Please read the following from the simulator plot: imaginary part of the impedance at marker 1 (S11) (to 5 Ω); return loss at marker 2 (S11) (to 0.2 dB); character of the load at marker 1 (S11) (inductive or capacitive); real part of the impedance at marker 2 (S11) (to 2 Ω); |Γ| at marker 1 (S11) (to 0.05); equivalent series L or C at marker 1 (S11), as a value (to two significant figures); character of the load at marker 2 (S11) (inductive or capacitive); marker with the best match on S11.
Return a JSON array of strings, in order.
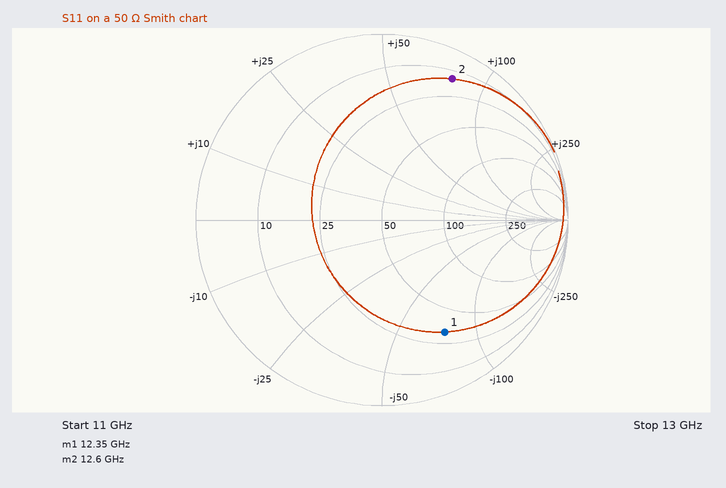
["-75 Ω", "1.4 dB", "capacitive", "14 Ω", "0.70", "170 fF", "inductive", "marker 1"]
